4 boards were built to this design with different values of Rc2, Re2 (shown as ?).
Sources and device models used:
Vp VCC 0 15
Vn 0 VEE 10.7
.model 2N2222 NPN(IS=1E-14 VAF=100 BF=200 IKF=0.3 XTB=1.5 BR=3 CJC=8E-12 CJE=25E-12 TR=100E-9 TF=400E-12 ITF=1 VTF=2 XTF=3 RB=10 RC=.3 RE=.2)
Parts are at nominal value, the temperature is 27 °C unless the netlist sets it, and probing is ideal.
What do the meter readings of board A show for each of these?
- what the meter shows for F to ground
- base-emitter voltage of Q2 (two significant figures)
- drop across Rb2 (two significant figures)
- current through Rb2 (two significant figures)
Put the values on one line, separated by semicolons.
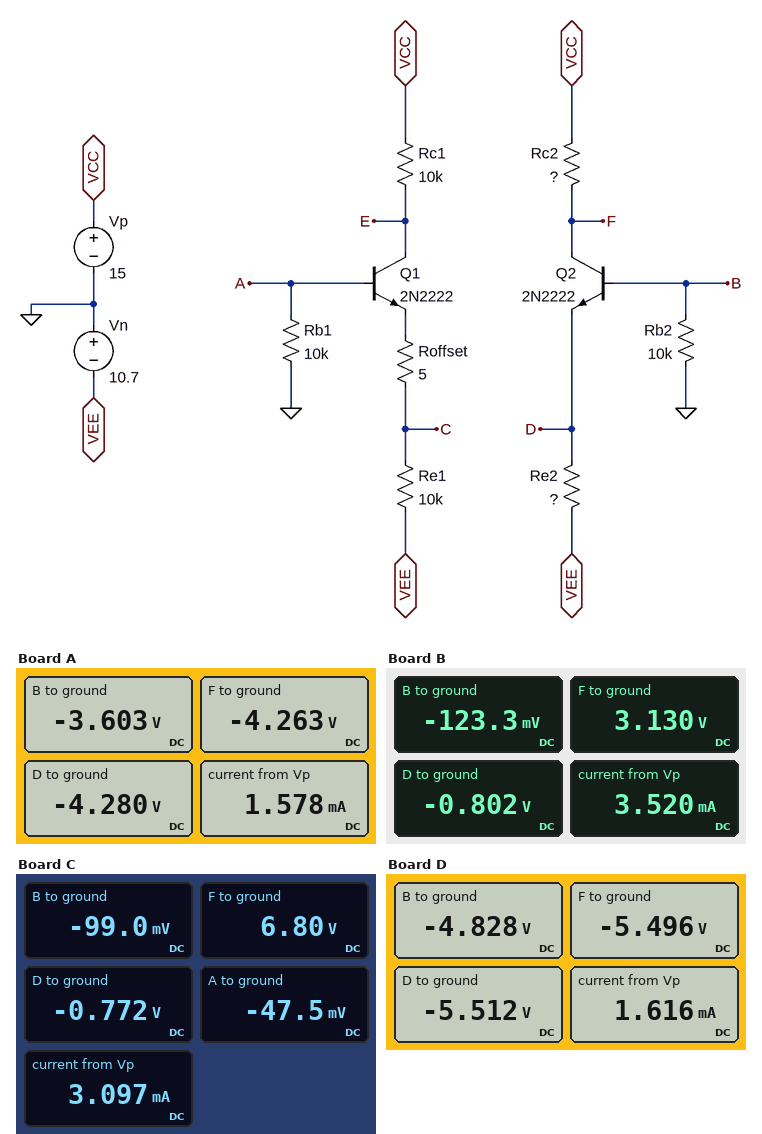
-4.263 V; 680 mV; 3.6 V; 360 µA
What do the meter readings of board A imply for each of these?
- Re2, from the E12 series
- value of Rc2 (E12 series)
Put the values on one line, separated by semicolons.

6.8 kΩ; 33 kΩ
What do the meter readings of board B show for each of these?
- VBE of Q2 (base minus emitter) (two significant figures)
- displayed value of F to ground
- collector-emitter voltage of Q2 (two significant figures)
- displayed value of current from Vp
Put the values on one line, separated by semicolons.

680 mV; 3.130 V; 3.9 V; 3.520 mA
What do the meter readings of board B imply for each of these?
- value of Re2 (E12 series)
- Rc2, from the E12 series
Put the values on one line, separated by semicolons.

3.9 kΩ; 4.7 kΩ
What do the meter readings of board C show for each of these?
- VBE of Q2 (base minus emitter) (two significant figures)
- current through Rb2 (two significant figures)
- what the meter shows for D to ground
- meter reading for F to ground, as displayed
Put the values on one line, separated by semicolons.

670 mV; 9.9 µA; -0.772 V; 6.80 V
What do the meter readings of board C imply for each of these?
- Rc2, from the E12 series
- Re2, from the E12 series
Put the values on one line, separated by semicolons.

3.9 kΩ; 4.7 kΩ
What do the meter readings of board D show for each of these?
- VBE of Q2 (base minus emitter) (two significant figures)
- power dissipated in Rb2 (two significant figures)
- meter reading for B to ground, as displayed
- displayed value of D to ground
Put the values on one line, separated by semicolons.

680 mV; 2.3 mW; -4.828 V; -5.512 V
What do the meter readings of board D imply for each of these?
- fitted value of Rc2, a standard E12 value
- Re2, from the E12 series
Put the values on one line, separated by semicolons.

33 kΩ; 4.7 kΩ
